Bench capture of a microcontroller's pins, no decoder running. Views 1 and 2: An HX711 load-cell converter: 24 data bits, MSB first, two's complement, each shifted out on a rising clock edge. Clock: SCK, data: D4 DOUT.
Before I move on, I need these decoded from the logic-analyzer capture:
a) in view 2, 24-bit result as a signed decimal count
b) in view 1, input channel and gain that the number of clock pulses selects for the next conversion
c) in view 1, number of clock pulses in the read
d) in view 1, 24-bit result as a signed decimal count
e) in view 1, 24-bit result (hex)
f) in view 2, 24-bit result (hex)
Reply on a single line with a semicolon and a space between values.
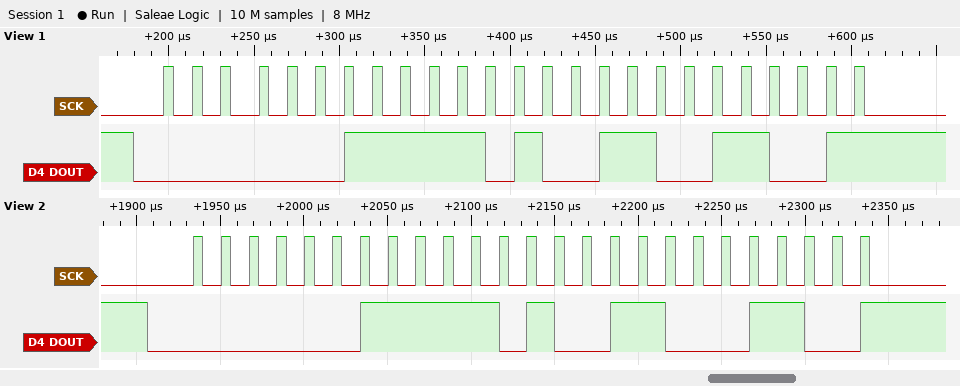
256396; channel A, gain 128; 25; 256409; 0x03E999; 0x03E98C
